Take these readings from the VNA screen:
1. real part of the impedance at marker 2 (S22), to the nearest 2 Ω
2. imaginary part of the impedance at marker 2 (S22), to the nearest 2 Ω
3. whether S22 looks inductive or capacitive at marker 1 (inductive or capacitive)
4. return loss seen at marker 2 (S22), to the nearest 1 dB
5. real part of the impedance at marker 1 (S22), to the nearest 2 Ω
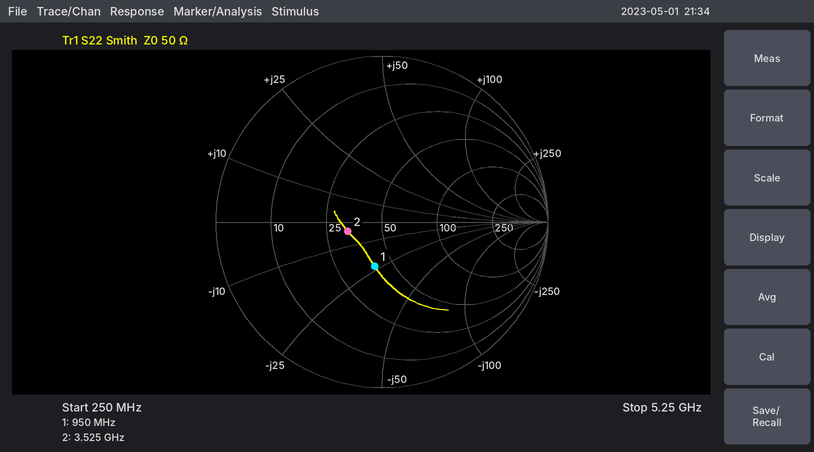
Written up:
32 Ω
-4 Ω
capacitive
13 dB
40 Ω
